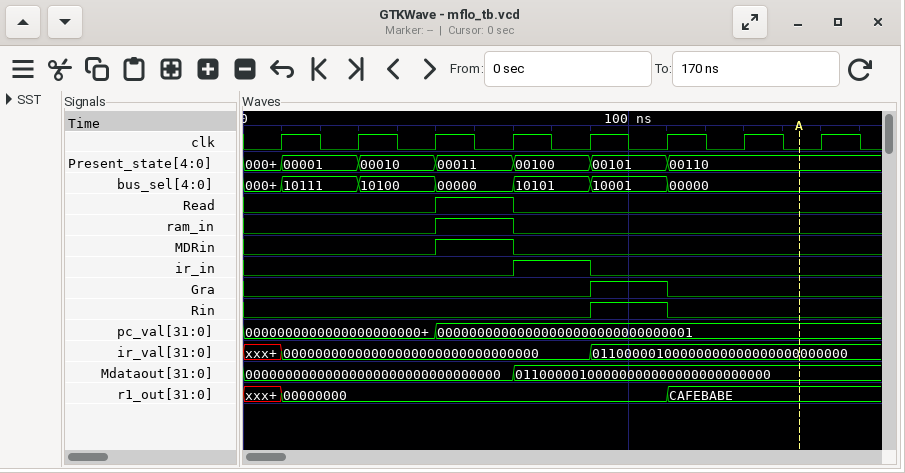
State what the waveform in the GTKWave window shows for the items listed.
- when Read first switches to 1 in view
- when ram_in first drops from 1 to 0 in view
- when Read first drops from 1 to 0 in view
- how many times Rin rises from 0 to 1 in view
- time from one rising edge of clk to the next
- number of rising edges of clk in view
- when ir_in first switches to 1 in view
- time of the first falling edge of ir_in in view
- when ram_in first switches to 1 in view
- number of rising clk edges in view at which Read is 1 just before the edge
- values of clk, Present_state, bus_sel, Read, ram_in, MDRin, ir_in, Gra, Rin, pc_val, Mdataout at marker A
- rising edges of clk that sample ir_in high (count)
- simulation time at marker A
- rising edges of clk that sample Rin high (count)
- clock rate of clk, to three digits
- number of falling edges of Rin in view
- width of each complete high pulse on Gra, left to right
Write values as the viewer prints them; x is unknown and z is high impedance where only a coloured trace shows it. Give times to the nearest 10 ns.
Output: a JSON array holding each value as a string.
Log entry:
["50 ns", "70 ns", "70 ns", "1", "20 ns", "8", "70 ns", "90 ns", "50 ns", "1", "clk=0, Present_state=00110, bus_sel=00000, Read=0, ram_in=0, MDRin=0, ir_in=0, Gra=0, Rin=0, pc_val=00000000000000000000000000000001, Mdataout=01100000100000000000000000000000", "1", "140 ns", "1", "50.0 MHz", "1", "20 ns"]
